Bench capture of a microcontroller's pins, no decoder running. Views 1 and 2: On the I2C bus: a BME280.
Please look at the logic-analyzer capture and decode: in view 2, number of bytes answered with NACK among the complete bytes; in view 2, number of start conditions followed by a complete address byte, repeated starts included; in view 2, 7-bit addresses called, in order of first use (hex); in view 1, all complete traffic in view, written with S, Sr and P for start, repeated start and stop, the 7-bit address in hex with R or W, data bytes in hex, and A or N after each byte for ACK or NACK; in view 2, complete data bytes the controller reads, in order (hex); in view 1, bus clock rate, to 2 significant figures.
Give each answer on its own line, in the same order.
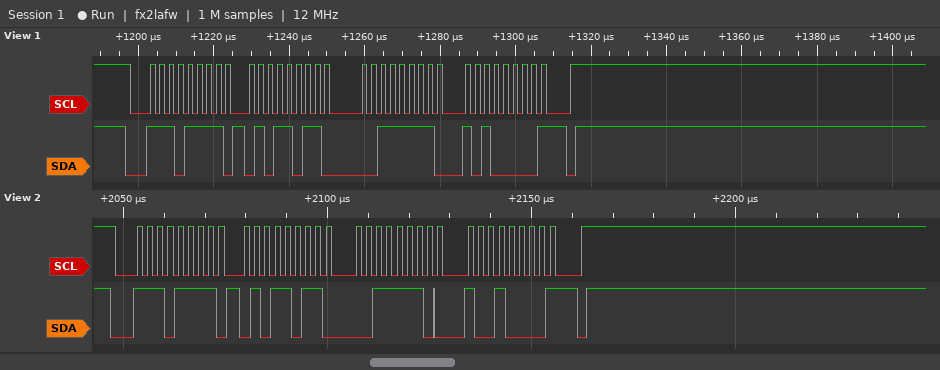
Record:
1
1
0x77
S 77R A 5B A 3F A A0 N P
5B 3E 90
400 kHz
